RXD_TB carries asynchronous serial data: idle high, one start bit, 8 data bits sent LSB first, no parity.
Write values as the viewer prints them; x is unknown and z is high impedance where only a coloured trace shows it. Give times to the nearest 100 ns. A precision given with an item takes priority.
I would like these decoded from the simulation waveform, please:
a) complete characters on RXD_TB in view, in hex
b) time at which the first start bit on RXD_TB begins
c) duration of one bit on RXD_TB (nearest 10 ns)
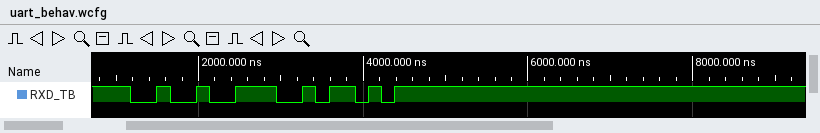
92, 5A
1200 ns
160 ns
